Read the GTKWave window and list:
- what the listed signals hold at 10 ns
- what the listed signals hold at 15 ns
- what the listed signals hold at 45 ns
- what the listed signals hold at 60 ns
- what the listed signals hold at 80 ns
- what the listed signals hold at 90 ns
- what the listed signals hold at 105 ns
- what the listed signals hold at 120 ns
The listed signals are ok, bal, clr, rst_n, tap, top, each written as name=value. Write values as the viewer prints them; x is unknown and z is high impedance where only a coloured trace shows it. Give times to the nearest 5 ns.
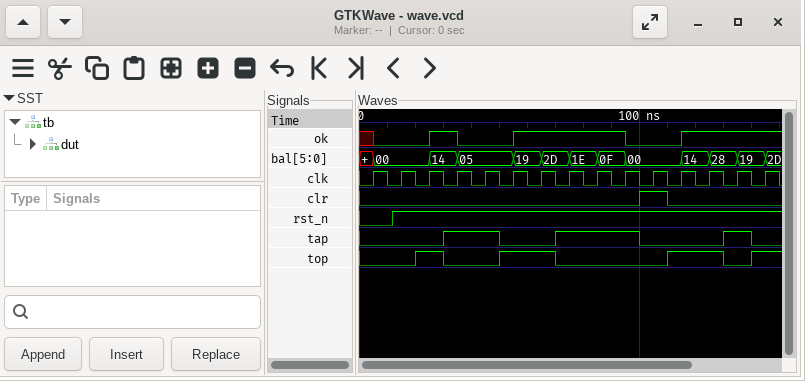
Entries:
ok=0, bal=00, clr=0, rst_n=0, tap=0, top=0
ok=0, bal=00, clr=0, rst_n=1, tap=0, top=0
ok=0, bal=05, clr=0, rst_n=1, tap=1, top=0
ok=1, bal=19, clr=0, rst_n=1, tap=0, top=1
ok=1, bal=1E, clr=0, rst_n=1, tap=1, top=0
ok=1, bal=0F, clr=0, rst_n=1, tap=1, top=0
ok=0, bal=00, clr=1, rst_n=1, tap=0, top=0
ok=1, bal=14, clr=0, rst_n=1, tap=0, top=1
